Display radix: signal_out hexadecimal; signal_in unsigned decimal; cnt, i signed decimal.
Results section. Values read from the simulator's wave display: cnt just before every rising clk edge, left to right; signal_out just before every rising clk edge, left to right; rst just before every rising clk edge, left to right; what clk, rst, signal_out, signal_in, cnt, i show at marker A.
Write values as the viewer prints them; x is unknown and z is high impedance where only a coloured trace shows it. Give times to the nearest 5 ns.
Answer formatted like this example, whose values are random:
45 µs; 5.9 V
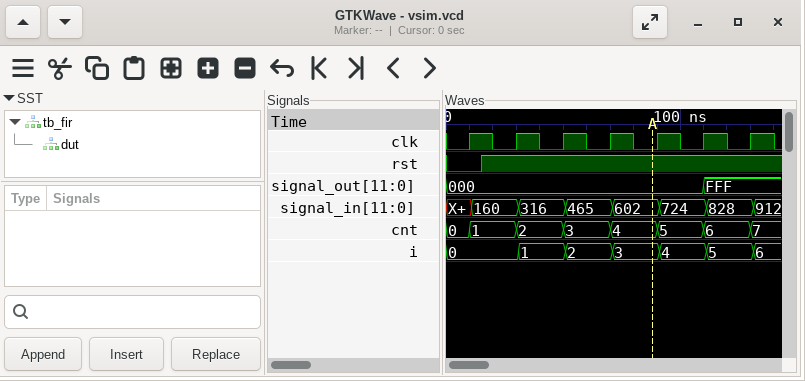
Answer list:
0, 1, 2, 3, 4, 5, 6; 000, 000, 000, 000, 000, 000, FFF; 0 1 1 1 1 1 1; clk=0, rst=1, signal_out=000, signal_in=602, cnt=4, i=3
